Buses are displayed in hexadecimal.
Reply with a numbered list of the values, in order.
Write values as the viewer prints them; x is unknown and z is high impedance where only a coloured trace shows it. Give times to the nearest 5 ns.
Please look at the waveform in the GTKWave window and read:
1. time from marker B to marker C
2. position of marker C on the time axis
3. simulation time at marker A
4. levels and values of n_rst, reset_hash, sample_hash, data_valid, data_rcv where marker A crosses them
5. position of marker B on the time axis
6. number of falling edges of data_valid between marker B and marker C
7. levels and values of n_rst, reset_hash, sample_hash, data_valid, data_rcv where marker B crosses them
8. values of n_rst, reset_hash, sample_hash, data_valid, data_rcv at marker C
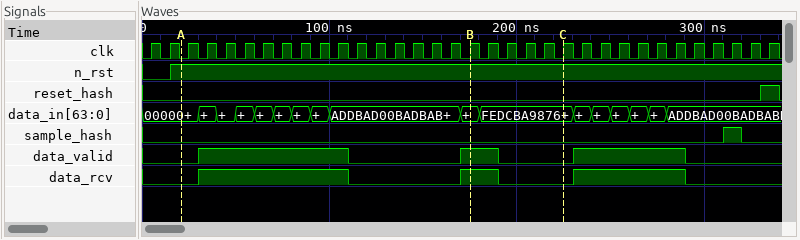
1. 50 ns
2. 225 ns
3. 20 ns
4. n_rst=1, reset_hash=0, sample_hash=0, data_valid=0, data_rcv=0
5. 175 ns
6. 1
7. n_rst=1, reset_hash=0, sample_hash=0, data_valid=1, data_rcv=1
8. n_rst=1, reset_hash=0, sample_hash=0, data_valid=0, data_rcv=0
